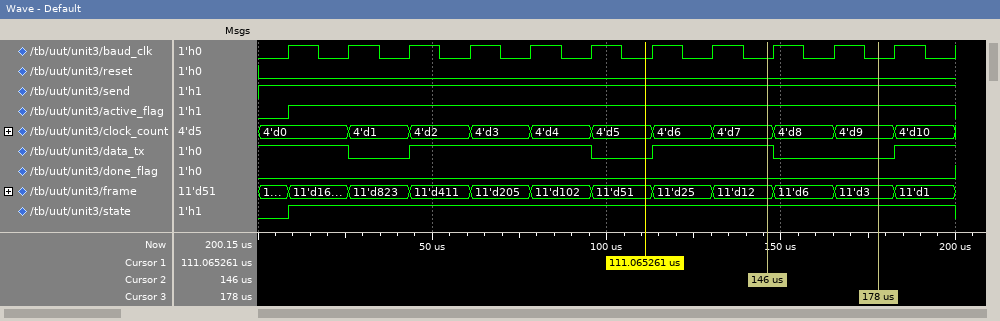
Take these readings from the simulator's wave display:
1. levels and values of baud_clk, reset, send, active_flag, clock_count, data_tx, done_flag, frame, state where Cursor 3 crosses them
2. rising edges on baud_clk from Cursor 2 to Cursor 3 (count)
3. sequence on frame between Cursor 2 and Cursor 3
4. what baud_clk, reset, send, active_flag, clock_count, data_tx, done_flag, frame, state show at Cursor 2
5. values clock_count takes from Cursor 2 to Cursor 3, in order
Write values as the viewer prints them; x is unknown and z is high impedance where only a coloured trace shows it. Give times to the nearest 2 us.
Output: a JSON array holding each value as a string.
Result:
["baud_clk=0, reset=0, send=1, active_flag=1, clock_count=4'd9, data_tx=0, done_flag=0, frame=11'd3, state=1", "2", "11'd12, 11'd6, 11'd3", "baud_clk=0, reset=0, send=1, active_flag=1, clock_count=4'd7, data_tx=1, done_flag=0, frame=11'd12, state=1", "4'd7, 4'd8, 4'd9"]
